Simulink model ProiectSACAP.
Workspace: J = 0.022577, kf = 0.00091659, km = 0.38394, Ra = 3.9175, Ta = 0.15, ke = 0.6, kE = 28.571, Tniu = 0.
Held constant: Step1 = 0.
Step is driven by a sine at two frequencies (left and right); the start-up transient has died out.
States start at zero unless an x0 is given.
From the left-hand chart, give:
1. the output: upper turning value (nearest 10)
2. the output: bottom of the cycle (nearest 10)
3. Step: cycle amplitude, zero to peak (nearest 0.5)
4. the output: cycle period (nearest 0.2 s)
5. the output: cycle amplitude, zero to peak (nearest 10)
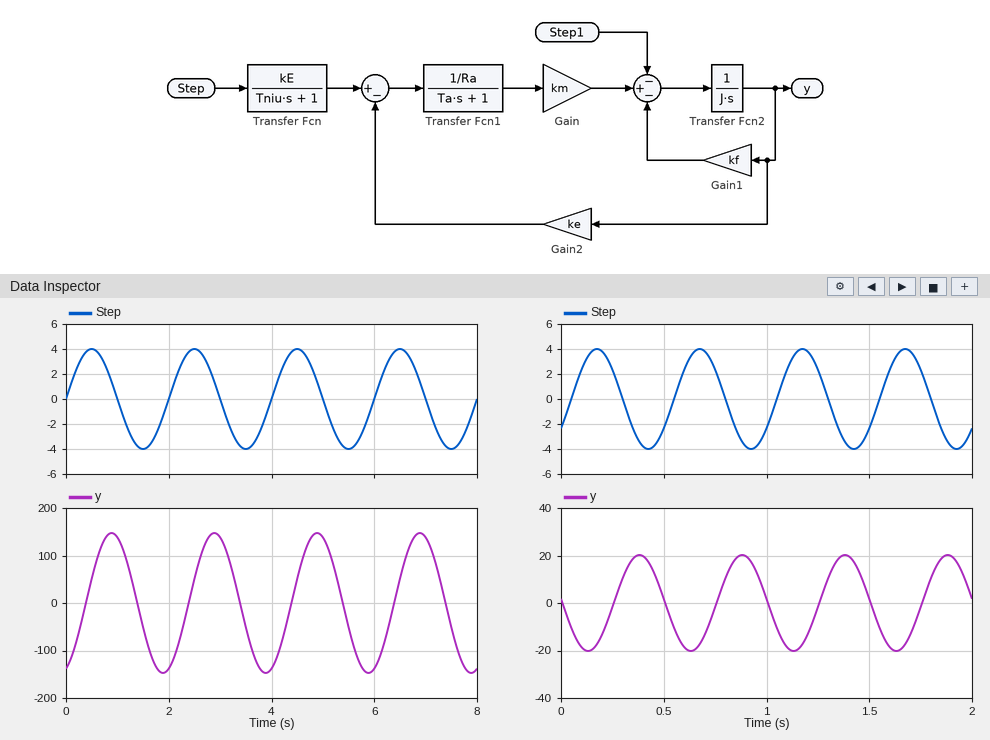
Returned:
150
-150
4.0
2.0 s
150
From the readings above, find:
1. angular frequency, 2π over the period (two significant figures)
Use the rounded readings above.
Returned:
3.1 rad/s
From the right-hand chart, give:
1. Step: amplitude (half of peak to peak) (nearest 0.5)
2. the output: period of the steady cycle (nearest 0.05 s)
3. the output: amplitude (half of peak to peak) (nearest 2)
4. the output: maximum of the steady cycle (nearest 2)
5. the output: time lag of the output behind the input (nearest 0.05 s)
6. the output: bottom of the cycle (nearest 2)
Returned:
4.0
0.50 s
20
20
0.20 s
-20
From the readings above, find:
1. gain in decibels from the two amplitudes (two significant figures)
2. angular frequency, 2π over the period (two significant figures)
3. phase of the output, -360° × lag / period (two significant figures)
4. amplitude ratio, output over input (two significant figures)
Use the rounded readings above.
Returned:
14 dB
13 rad/s
-140°
5.0
